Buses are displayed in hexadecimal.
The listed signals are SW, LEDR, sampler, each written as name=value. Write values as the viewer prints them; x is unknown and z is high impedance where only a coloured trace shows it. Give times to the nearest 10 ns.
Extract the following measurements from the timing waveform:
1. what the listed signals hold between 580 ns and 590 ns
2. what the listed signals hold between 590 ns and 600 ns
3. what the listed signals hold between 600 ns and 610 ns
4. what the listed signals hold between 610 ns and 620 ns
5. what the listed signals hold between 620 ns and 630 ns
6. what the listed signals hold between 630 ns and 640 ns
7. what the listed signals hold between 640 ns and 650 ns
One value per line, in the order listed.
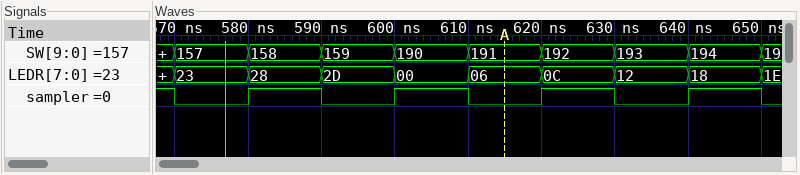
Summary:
SW=158, LEDR=28, sampler=1
SW=159, LEDR=2D, sampler=0
SW=190, LEDR=00, sampler=1
SW=191, LEDR=06, sampler=0
SW=192, LEDR=0C, sampler=1
SW=193, LEDR=12, sampler=0
SW=194, LEDR=18, sampler=1
